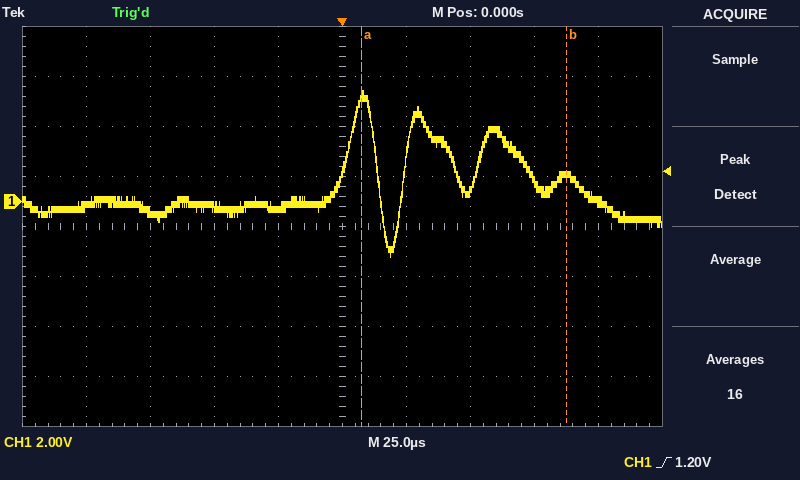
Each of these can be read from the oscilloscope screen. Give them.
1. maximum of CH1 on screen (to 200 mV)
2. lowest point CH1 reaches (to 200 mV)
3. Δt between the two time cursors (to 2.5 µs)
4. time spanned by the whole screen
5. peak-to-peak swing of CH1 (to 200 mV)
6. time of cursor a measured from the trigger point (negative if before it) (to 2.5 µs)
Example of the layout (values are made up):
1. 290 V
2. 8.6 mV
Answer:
1. 4.4 V
2. -2.2 V
3. 80.0 µs
4. 250 µs
5. 6.6 V
6. +7.5 µs
